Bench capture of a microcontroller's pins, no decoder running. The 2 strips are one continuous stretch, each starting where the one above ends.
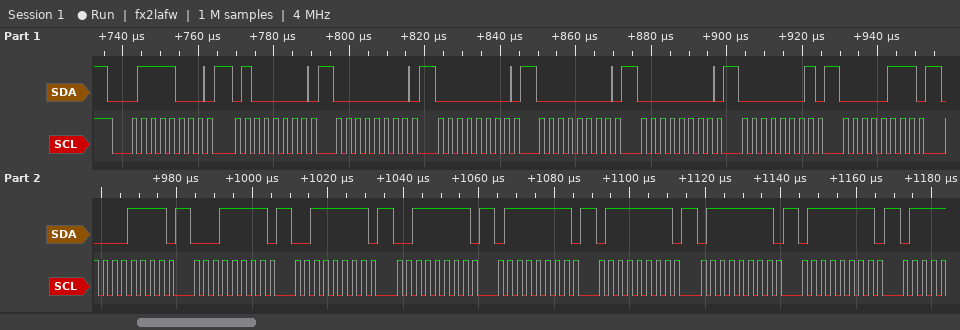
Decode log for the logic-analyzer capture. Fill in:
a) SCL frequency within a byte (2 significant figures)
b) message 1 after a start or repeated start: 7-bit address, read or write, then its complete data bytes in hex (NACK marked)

400 kHz
0x3C write: 40 00 00 00 00 01 07 0F 1F 3F 3F 7F 7F 7F 7F
